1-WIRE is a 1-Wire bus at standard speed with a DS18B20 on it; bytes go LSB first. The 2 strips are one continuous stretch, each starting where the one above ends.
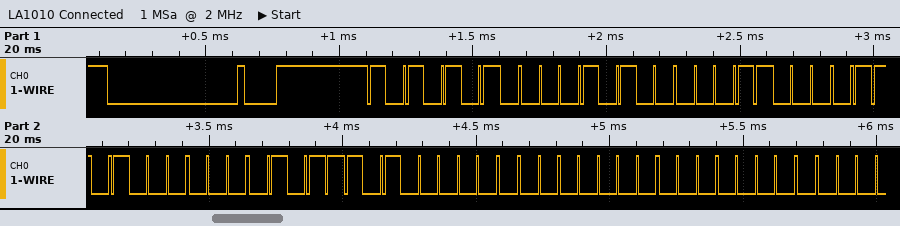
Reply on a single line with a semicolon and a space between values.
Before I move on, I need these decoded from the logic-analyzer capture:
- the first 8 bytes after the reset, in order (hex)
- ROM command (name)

55 28 18 16 D0 05 00 00; Match ROM
